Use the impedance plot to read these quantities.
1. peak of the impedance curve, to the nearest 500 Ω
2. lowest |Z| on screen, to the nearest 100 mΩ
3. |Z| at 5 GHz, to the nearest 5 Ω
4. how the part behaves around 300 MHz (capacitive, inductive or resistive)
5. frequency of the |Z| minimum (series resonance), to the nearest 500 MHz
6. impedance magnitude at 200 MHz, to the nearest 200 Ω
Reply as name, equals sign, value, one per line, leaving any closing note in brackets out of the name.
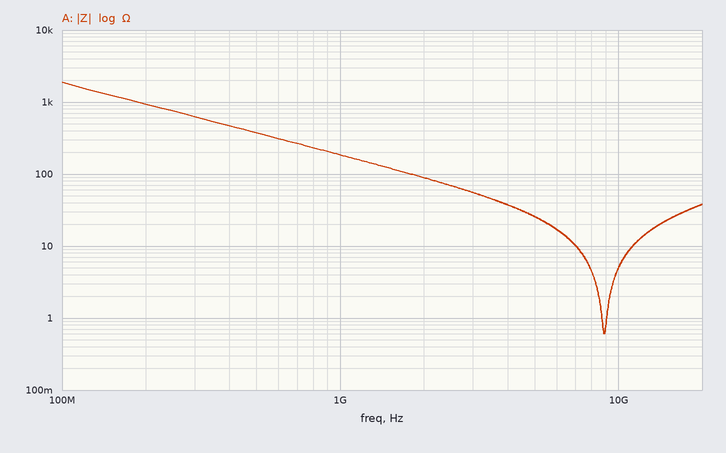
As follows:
peak of the impedance curve, to the nearest 500 Ω = 2.0 kΩ
lowest |Z| on screen, to the nearest 100 mΩ = 600 mΩ
|Z| at 5 GHz, to the nearest 5 Ω = 25 Ω
how the part behaves around 300 MHz = capacitive
frequency of the |Z| minimum (series resonance), to the nearest 500 MHz = 9.0 GHz
impedance magnitude at 200 MHz, to the nearest 200 Ω = 1.0 kΩ
